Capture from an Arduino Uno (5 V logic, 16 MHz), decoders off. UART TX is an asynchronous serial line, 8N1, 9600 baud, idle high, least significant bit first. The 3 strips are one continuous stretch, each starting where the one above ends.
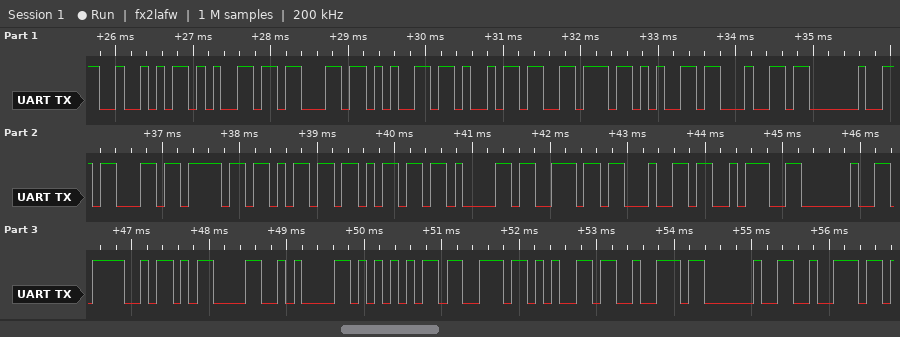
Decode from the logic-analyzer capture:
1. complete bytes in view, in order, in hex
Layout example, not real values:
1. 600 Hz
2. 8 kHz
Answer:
1. 0x52 0x65 0x63 0x65 0x69 0x76 0x65 0x64 0x20 0x63 0x6F 0x6D 0x6D 0x61 0x6E 0x64 0x3A 0x20 0x4F 0x0D 0x0A 0x55 0x73 0x65 0x72 0x20 0x72
